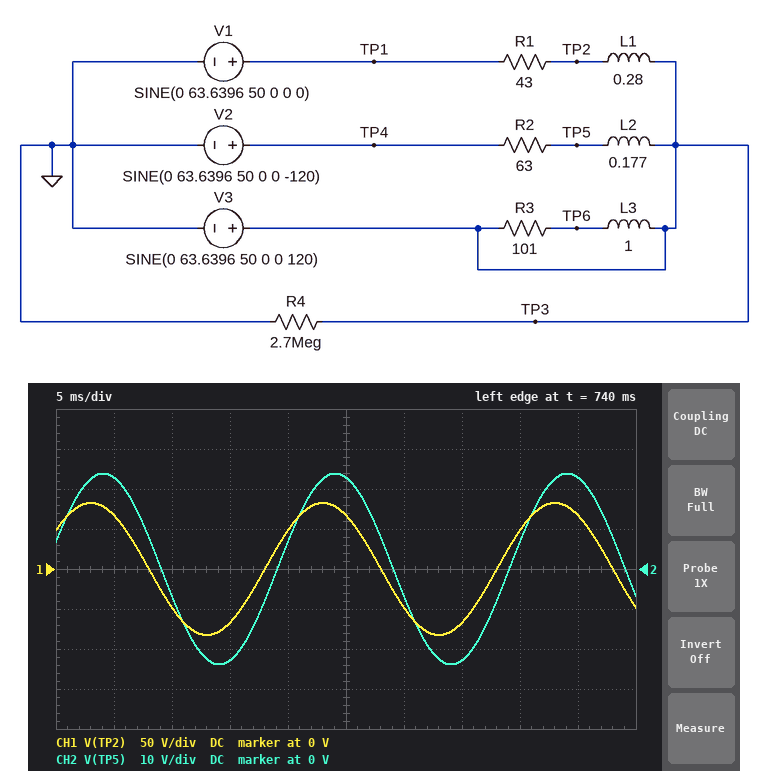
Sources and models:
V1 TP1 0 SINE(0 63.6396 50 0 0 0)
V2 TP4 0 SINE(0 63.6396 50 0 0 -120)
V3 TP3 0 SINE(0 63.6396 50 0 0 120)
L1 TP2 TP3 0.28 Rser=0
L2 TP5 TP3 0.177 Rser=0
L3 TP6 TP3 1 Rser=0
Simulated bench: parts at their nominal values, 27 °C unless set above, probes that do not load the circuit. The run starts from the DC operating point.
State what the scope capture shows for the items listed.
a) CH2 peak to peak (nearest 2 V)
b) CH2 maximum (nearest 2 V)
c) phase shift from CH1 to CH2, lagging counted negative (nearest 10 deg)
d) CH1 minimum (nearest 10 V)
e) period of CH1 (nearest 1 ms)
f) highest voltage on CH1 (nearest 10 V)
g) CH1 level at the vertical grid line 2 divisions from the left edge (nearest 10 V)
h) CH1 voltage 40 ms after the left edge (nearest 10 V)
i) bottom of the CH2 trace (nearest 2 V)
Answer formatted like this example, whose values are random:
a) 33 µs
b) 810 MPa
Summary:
a) 48 V
b) 24 V
c) -20 deg
d) -80 V
e) 20 ms
f) 80 V
g) -50 V
h) 50 V
i) -24 V
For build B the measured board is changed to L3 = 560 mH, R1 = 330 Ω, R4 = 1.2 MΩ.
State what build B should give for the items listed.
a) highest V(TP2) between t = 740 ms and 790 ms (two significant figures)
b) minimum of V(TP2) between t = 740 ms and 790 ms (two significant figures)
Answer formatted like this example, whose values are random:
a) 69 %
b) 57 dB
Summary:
a) 76 V
b) -76 V
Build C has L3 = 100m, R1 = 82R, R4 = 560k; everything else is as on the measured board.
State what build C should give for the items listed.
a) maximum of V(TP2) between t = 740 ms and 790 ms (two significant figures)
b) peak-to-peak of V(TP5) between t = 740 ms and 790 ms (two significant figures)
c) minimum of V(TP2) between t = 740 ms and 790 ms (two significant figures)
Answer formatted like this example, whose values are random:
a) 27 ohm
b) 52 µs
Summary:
a) 87 V
b) 48 V
c) -87 V
